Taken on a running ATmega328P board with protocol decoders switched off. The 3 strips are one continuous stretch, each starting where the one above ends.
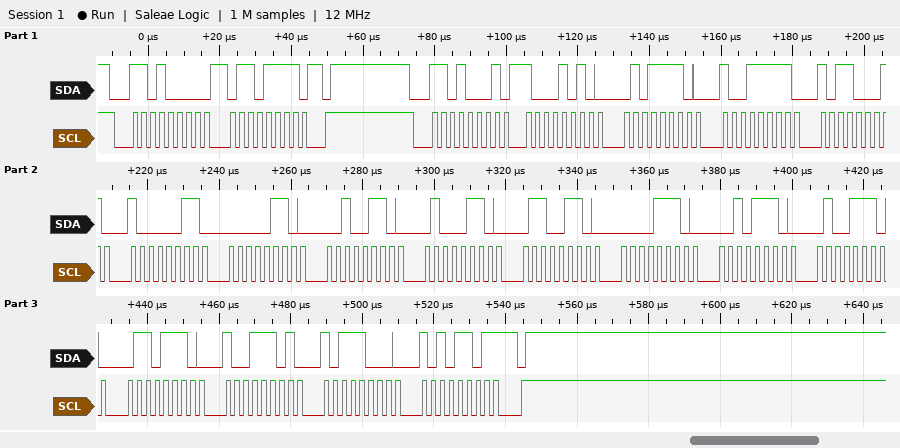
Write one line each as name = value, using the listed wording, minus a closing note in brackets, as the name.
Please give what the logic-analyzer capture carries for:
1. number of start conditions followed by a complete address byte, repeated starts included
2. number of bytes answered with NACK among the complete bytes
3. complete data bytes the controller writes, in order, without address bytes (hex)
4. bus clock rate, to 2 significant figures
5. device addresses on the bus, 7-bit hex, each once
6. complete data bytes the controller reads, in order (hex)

number of start conditions followed by a complete address byte, repeated starts included = 2
number of bytes answered with NACK among the complete bytes = 1
complete data bytes the controller writes, in order, without address bytes = 6F
bus clock rate, to 2 significant figures = 400 kHz
device addresses on the bus, 7-bit hex, each once = 0x68
complete data bytes the controller reads, in order = 8A 5E 9F B1 83 06 26 46 66 0E 2E 4E 6E 9D B8 AD
